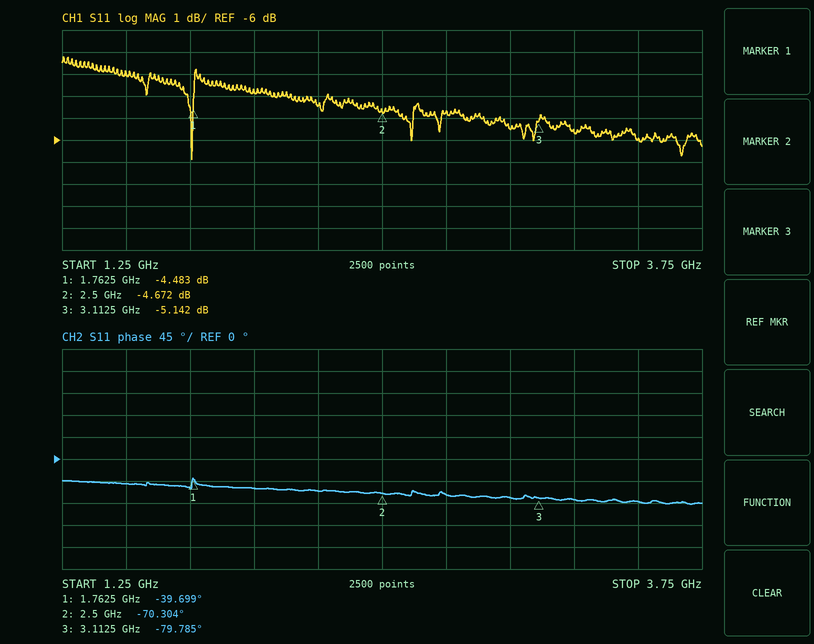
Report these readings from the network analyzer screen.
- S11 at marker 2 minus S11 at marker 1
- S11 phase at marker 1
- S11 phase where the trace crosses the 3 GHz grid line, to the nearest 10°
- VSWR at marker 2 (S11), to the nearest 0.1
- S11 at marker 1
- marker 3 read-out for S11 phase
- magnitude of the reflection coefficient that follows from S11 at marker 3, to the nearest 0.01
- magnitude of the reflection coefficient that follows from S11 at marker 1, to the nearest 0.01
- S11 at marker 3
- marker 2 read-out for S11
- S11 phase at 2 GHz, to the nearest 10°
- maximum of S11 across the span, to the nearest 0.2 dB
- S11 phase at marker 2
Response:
-0.189 dB
-39.699°
-80°
3.8
-4.483 dB
-79.785°
0.55
0.60
-5.142 dB
-4.672 dB
-60°
-2.2 dB
-70.304°
